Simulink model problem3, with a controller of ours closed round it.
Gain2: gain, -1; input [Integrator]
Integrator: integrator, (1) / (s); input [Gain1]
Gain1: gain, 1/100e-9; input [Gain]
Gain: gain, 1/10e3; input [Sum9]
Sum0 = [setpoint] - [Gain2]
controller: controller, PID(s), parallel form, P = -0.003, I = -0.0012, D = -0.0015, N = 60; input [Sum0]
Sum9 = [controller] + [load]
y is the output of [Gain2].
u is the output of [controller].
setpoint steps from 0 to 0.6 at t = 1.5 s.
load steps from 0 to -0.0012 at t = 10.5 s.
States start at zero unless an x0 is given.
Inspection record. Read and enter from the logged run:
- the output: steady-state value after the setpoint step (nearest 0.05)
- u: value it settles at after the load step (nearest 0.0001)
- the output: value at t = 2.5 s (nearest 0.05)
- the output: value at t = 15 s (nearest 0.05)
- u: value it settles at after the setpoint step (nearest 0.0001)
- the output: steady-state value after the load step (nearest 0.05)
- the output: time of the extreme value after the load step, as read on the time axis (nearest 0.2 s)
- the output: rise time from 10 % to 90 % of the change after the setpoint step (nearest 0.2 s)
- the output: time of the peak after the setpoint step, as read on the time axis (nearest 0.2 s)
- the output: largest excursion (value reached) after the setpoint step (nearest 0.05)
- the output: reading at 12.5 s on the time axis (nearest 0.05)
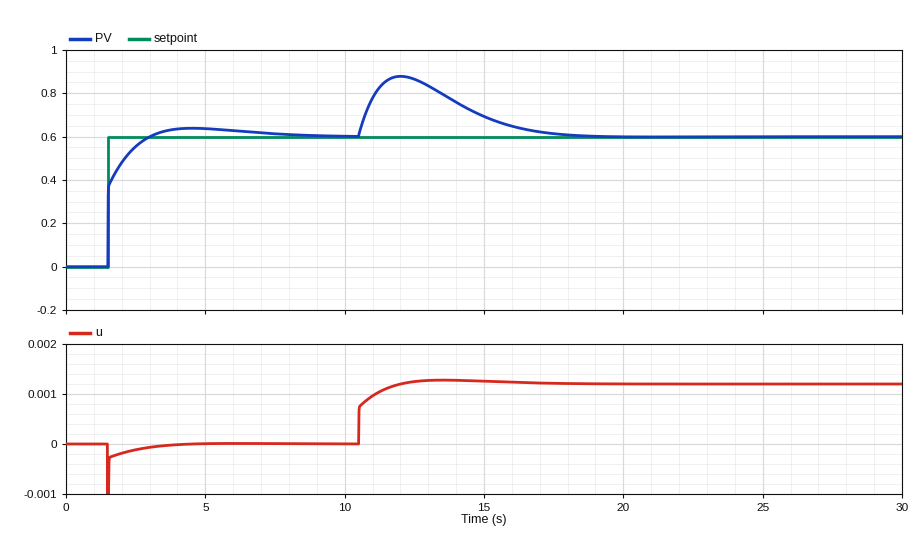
0.60
0.0012
0.55
0.70
0.0000
0.60
12.0 s
0.8 s
4.6 s
0.65
0.85
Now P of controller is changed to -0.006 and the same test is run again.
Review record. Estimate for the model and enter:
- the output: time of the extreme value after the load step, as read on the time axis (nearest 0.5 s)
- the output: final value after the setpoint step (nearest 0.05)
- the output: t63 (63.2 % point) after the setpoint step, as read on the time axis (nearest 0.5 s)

11.5 s
0.60
1.5 s
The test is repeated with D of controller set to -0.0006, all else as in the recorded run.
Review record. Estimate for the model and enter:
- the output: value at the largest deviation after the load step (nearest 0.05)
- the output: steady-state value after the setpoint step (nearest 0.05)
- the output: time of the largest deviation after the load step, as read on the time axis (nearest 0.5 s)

0.90
0.60
11.5 s
